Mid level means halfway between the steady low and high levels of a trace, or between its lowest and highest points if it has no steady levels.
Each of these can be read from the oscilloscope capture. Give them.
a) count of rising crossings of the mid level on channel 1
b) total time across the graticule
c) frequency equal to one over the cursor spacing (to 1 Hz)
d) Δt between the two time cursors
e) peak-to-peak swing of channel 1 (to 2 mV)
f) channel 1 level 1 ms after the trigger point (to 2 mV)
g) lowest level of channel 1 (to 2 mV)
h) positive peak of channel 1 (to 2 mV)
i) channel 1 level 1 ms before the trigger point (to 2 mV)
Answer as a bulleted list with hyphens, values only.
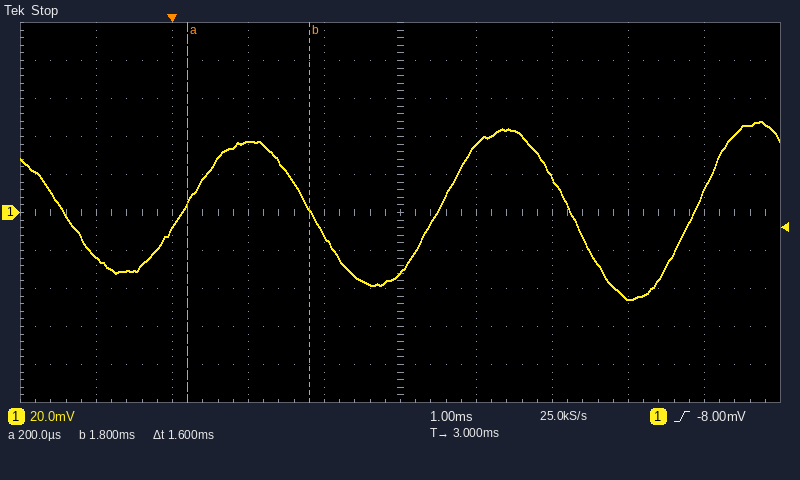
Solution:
- 3
- 10 ms
- 625 Hz
- 1.6 ms
- 94 mV
- 38 mV
- -46 mV
- 48 mV
- -24 mV
